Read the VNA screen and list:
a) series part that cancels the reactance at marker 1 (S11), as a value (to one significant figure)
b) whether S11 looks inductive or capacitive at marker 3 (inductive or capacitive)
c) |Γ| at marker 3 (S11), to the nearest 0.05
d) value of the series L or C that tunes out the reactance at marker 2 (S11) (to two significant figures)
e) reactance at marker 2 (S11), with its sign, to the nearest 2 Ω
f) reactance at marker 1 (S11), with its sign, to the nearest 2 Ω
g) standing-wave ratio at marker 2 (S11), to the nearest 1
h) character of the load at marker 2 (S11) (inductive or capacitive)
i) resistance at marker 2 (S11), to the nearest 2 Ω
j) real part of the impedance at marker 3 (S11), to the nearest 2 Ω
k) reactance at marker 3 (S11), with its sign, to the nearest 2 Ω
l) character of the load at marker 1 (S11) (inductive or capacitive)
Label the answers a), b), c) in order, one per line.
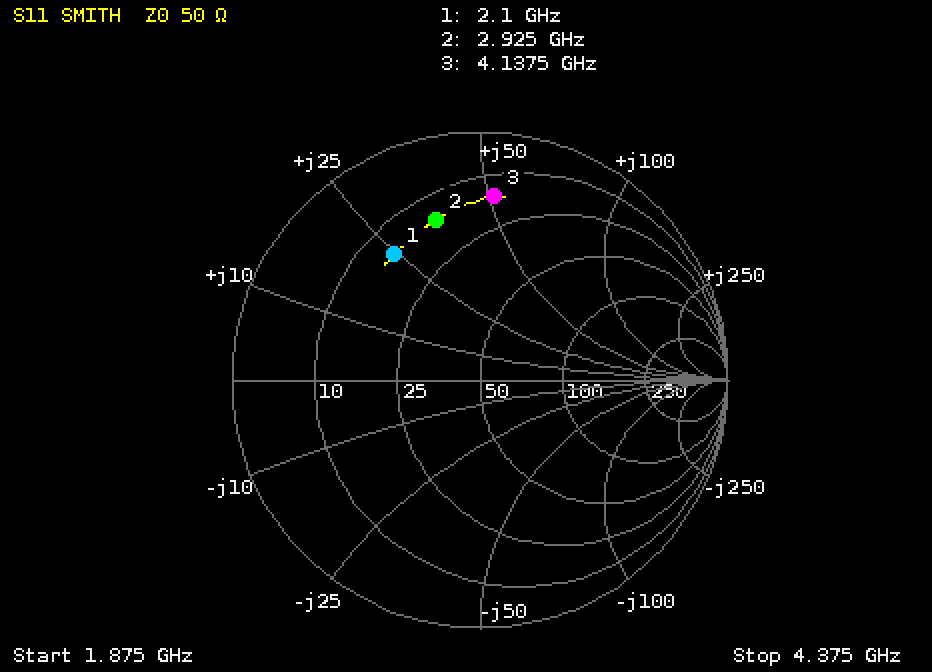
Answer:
a) 3 pF
b) inductive
c) 0.75
d) 1.5 pF
e) +36 Ω
f) +24 Ω
g) 5
h) inductive
i) 16 Ω
j) 16 Ω
k) +52 Ω
l) inductive
